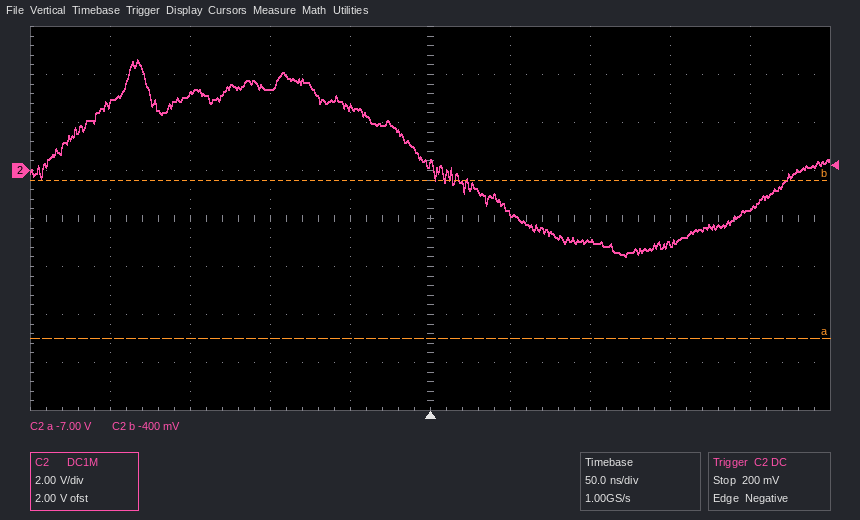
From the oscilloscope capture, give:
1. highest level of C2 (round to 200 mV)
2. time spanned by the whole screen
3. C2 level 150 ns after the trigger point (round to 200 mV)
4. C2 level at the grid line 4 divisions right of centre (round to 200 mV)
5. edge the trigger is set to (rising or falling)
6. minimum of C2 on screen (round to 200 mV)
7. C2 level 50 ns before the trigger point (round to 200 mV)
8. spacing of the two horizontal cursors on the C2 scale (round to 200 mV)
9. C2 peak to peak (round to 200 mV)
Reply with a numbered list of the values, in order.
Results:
1. 4.6 V
2. 500 ns
3. -3.0 V
4. -1.6 V
5. falling
6. -3.6 V
7. 2.6 V
8. 6.6 V
9. 8.2 V
